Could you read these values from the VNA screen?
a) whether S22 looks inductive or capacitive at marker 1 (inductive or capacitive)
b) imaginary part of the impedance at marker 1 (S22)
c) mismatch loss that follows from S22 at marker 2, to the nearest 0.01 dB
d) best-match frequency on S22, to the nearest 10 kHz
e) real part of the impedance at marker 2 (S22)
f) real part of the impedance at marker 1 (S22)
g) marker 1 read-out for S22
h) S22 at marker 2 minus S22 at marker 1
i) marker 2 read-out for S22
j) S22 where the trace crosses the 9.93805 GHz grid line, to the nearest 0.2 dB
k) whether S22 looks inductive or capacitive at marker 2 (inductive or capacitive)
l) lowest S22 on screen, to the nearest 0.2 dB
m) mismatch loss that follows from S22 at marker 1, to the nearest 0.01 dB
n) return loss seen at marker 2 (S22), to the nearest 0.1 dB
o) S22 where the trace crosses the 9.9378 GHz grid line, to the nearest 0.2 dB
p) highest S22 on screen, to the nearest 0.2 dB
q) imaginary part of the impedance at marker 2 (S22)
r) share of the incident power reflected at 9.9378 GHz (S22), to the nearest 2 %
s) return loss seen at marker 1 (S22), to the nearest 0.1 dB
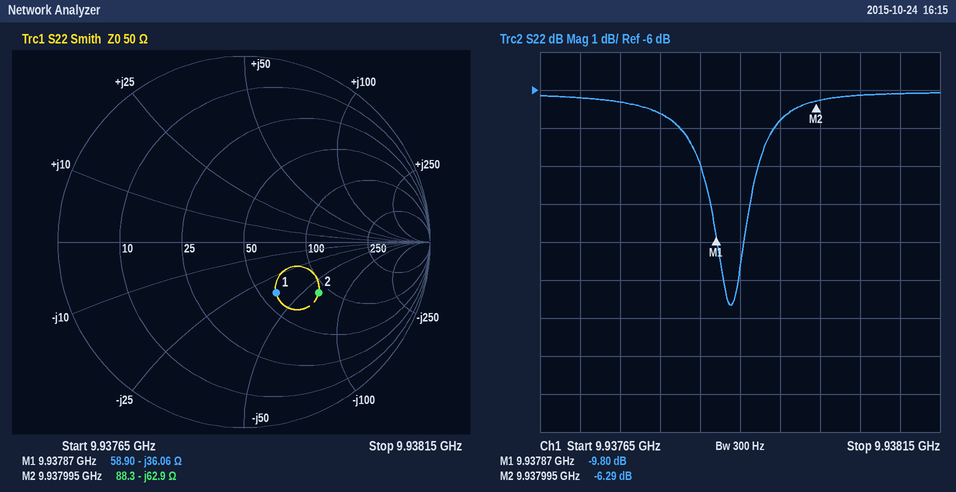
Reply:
capacitive
-36.06 Ω
1.16 dB
9.93789 GHz
88.3 Ω
58.90 Ω
-9.80 dB
3.51 dB
-6.29 dB
-6.2 dB
capacitive
-11.6 dB
0.48 dB
6.3 dB
-6.6 dB
-6.0 dB
-62.9 Ω
22 %
9.8 dB
